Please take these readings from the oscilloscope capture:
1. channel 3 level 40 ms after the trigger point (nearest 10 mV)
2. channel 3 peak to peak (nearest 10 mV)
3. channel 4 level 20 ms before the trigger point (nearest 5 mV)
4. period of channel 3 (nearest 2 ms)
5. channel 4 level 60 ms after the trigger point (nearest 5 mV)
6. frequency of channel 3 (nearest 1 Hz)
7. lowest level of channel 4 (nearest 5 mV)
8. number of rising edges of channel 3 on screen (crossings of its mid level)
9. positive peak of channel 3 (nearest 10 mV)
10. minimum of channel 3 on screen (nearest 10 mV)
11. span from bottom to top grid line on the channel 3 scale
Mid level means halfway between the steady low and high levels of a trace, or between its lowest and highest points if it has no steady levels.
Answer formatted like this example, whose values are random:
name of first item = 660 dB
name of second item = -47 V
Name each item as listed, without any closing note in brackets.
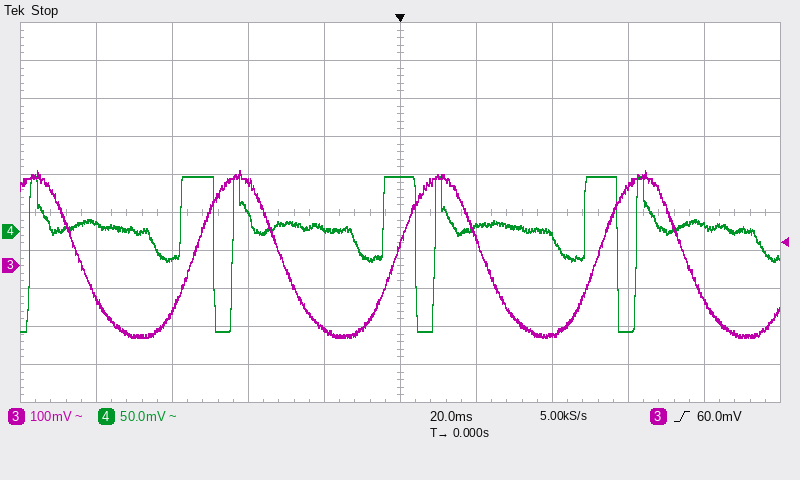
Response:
channel 3 level 40 ms after the trigger point = -180 mV
channel 3 peak to peak = 440 mV
channel 4 level 20 ms before the trigger point = 5 mV
period of channel 3 = 54 ms
channel 4 level 60 ms after the trigger point = -130 mV
frequency of channel 3 = 19 Hz
lowest level of channel 4 = -130 mV
number of rising edges of channel 3 on screen = 3
positive peak of channel 3 = 250 mV
minimum of channel 3 on screen = -190 mV
span from bottom to top grid line on the channel 3 scale = 1 V
